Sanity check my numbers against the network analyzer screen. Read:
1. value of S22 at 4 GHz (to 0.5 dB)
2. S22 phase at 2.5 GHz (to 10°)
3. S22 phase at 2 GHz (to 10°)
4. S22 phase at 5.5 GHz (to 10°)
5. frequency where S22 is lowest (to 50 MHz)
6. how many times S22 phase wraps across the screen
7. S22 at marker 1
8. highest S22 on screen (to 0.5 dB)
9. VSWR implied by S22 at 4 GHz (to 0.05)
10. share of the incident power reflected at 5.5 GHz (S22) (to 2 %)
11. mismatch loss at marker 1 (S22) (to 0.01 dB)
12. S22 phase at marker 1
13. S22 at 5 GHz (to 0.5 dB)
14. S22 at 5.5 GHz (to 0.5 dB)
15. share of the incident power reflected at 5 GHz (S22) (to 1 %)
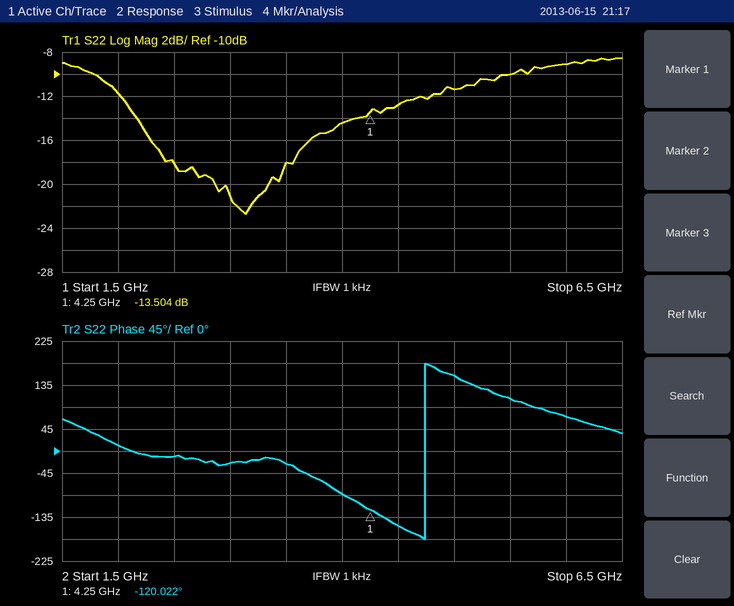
-14.5 dB
-10°
10°
110°
3.15 GHz
1
-13.504 dB
-8.5 dB
1.45
10 %
0.20 dB
-120.022°
-11.5 dB
-10.0 dB
7 %
